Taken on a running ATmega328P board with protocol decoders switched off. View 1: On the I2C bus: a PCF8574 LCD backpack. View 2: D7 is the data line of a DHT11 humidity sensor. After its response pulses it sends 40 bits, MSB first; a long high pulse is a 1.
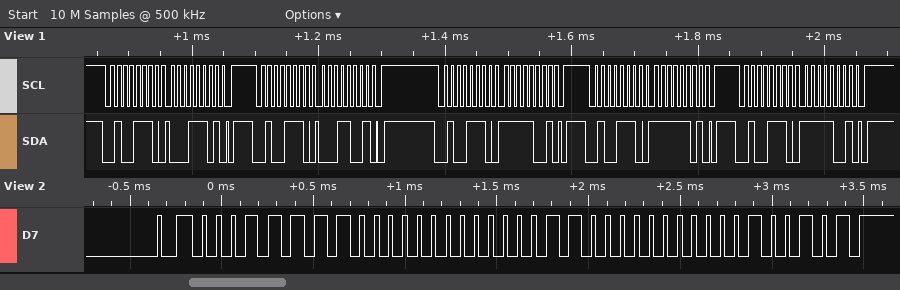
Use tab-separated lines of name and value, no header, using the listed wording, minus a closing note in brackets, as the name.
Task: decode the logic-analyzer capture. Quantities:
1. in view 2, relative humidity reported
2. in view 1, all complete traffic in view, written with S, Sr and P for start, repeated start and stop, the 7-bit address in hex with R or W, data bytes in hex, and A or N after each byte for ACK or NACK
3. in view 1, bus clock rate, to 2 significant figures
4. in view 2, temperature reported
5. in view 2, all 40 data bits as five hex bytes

in view 2, relative humidity reported	31 %
in view 1, all complete traffic in view, written with S, Sr and P for start, repeated start and stop, the 7-bit address in hex with R or W, data bytes in hex, and A or N after each byte for ACK or NACK	S 27W A 1D A P S 27W A 19 A P S 27W A F9 A P S 27W A FD A P S 27W A F9 A P
in view 1, bus clock rate, to 2 significant figures	100 kHz
in view 2, temperature reported	6.0 °C
in view 2, all 40 data bits as five hex bytes	1F 00 06 00 25
